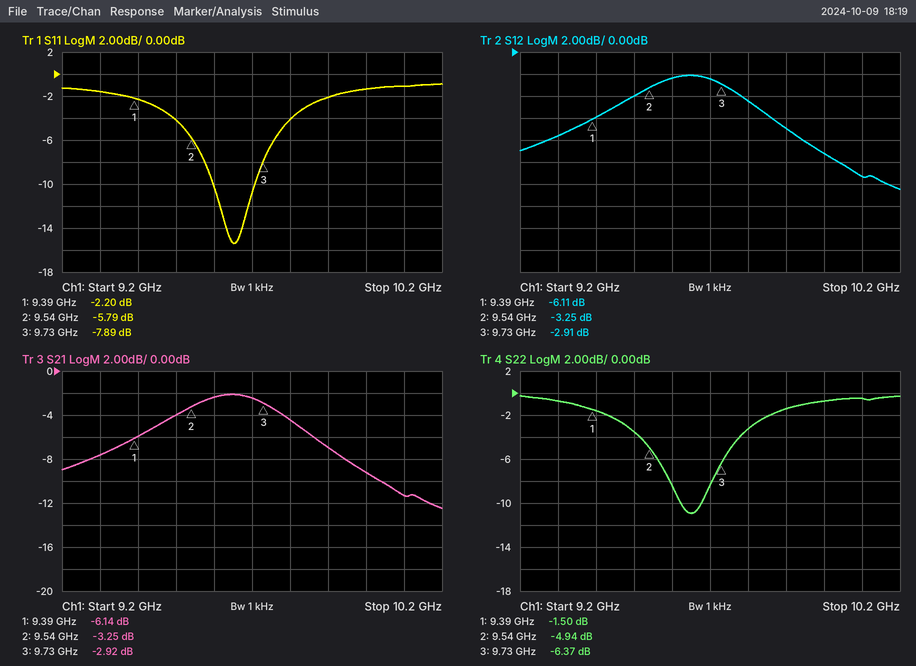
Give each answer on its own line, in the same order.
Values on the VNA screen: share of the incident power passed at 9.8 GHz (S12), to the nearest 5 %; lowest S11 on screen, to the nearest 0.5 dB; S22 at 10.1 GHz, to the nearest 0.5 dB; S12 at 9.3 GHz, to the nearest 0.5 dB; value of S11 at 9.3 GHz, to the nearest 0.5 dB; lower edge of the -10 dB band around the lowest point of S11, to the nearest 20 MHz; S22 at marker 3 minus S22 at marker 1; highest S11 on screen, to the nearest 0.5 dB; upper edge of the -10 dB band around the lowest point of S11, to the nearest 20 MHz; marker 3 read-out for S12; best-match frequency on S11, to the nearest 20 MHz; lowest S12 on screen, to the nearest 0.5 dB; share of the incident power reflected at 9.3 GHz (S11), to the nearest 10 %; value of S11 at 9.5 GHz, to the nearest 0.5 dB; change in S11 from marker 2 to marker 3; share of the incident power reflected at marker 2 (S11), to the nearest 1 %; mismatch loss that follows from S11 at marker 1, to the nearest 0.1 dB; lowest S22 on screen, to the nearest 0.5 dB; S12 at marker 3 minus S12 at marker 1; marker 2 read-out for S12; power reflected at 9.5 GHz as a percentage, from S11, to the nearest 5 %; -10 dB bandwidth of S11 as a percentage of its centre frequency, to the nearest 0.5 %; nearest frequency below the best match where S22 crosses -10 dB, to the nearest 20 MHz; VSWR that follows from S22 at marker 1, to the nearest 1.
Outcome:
35 %
-15.5 dB
-0.5 dB
-7.5 dB
-1.5 dB
9.60 GHz
-4.87 dB
-1.0 dB
9.70 GHz
-2.91 dB
9.66 GHz
-12.5 dB
70 %
-4.0 dB
-2.10 dB
26 %
4.0 dB
-11.0 dB
3.20 dB
-3.25 dB
40 %
1.0 %
9.62 GHz
12
